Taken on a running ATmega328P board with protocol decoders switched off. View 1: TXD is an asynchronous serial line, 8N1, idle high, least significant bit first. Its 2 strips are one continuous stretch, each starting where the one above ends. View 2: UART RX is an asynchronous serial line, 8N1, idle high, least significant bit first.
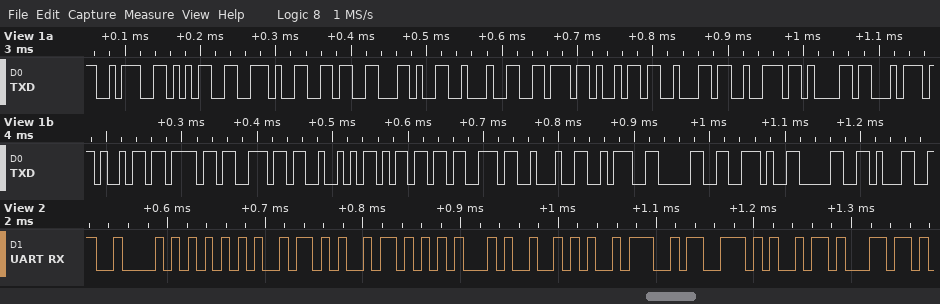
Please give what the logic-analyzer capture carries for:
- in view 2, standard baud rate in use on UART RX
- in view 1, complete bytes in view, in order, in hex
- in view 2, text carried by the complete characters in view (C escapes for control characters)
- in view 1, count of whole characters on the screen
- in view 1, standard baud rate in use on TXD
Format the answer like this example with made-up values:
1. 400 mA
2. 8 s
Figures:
1. 115200 baud
2. 3A 35 2E 36 2C 22 76 69 62 72 61 74 69 6F 6E 52 6D 73 22 3A 30 2E 30 31
3. "BUZZER:sil"
4. 24
5. 115200 baud
